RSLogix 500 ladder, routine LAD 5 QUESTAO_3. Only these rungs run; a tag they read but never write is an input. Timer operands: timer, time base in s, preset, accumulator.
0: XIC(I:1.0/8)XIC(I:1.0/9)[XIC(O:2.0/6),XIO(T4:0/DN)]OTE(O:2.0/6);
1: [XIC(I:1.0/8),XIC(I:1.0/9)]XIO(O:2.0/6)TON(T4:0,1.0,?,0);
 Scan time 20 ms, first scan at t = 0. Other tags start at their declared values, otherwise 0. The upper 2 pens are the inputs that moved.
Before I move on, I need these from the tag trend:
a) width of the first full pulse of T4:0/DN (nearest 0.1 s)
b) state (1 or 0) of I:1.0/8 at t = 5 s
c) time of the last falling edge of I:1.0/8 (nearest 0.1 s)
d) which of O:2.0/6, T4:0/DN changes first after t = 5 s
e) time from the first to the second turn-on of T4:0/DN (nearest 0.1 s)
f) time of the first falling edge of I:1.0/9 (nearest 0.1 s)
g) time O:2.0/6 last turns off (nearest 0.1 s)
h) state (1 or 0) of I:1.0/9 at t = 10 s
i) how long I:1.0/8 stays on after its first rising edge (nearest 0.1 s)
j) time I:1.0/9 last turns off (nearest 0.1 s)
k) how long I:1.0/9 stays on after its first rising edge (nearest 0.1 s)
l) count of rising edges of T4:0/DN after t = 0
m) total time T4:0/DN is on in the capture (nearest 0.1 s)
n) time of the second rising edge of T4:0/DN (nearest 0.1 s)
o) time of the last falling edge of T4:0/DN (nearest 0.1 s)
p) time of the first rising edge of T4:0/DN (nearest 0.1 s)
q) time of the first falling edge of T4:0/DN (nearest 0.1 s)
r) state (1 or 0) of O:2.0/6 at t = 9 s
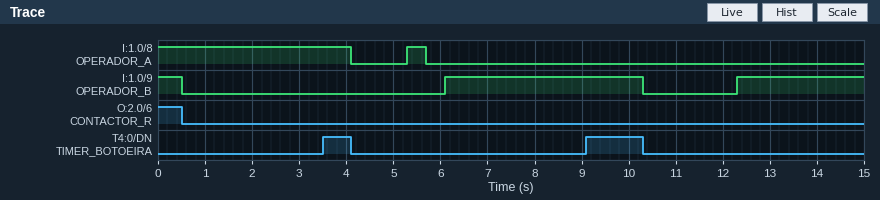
0.6 s
0
5.7 s
T4:0/DN
5.6 s
0.5 s
0.5 s
1
0.4 s
10.3 s
4.2 s
2
1.8 s
9.1 s
10.3 s
3.5 s
4.1 s
0
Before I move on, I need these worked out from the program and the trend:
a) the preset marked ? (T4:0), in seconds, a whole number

3 s
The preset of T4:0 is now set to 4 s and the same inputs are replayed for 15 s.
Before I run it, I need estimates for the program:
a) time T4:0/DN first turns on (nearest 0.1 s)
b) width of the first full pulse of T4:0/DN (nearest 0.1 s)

10.1 s
0.2 s
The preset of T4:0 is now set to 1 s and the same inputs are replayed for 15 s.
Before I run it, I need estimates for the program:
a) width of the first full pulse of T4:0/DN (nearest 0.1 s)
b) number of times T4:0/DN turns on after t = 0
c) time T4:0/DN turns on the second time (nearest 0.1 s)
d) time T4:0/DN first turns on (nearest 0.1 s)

2.6 s
3
7.1 s
1.5 s
